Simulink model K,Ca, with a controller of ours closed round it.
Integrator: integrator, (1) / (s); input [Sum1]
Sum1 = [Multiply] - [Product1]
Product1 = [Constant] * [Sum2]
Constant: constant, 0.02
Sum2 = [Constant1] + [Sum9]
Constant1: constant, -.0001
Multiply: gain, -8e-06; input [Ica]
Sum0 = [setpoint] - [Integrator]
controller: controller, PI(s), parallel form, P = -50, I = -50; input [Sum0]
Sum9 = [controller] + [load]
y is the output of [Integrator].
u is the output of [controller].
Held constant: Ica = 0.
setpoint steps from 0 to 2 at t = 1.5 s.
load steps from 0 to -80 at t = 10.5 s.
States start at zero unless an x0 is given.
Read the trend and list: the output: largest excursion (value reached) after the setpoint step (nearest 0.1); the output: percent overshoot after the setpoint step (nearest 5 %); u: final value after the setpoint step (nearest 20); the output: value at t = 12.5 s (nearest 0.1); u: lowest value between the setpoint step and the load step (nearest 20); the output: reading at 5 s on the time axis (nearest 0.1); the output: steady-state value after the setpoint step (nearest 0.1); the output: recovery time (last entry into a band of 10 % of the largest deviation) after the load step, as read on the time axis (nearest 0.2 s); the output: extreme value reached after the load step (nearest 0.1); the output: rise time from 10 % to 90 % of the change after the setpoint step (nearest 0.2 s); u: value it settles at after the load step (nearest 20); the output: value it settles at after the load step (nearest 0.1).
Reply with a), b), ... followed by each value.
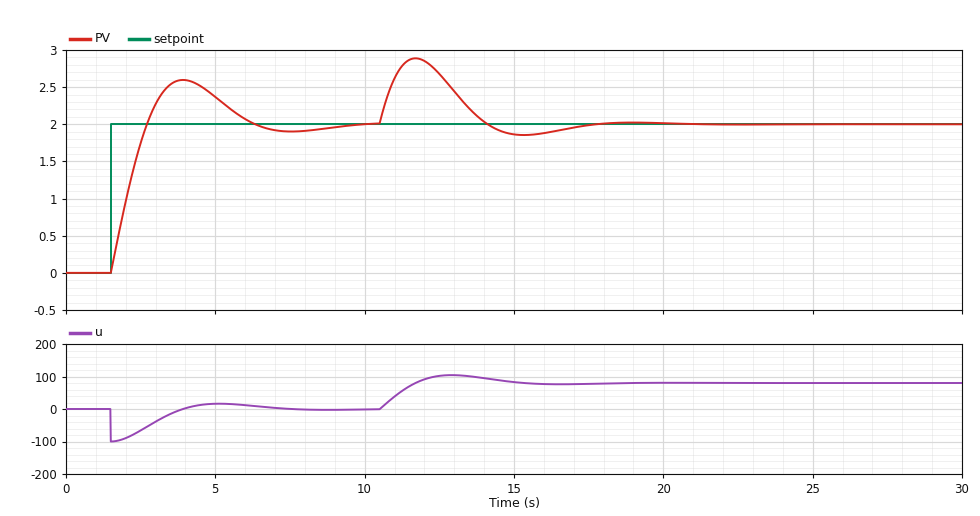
a) 2.6
b) 30 %
c) 0
d) 2.7
e) -100
f) 2.4
g) 2.0
h) 16.4 s
i) 2.9
j) 1.0 s
k) 80
l) 2.0
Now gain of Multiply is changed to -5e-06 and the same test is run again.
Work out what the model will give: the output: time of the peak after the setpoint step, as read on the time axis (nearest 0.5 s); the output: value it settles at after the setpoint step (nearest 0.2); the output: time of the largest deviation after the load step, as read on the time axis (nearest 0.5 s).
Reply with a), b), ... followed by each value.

a) 4.0 s
b) 2.0
c) 11.5 s
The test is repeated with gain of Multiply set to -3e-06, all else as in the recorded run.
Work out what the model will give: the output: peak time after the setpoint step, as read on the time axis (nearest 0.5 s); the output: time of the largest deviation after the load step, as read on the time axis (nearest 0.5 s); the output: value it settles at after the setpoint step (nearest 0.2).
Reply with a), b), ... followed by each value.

a) 4.0 s
b) 11.5 s
c) 2.0
